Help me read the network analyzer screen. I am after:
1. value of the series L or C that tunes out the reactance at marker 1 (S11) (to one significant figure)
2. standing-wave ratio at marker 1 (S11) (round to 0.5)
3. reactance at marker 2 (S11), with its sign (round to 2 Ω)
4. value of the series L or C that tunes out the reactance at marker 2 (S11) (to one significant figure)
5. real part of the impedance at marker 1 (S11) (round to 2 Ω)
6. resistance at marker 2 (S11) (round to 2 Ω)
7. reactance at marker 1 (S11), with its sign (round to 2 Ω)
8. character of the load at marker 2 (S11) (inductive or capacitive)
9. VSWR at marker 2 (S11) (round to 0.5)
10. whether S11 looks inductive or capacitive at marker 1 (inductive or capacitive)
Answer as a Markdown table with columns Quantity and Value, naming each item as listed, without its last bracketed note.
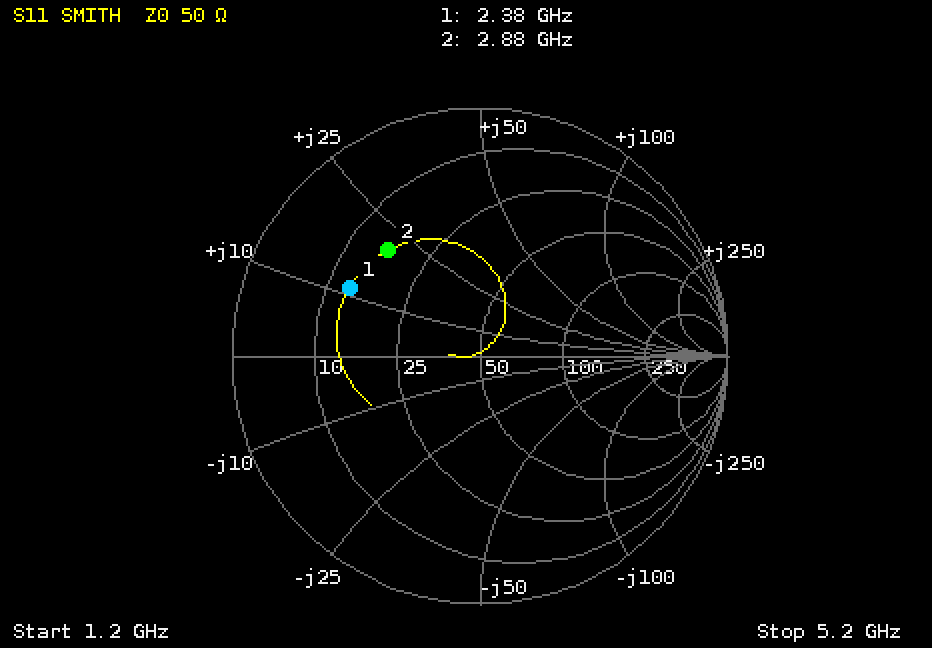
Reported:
| Quantity | Value |
|---|---|
| value of the series L or C that tunes out the reactance at marker 1 (S11) | 6 pF |
| standing-wave ratio at marker 1 (S11) | 4.0 |
| reactance at marker 2 (S11), with its sign | +20 Ω |
| value of the series L or C that tunes out the reactance at marker 2 (S11) | 3 pF |
| real part of the impedance at marker 1 (S11) | 14 Ω |
| resistance at marker 2 (S11) | 16 Ω |
| reactance at marker 1 (S11), with its sign | +12 Ω |
| character of the load at marker 2 (S11) | inductive |
| VSWR at marker 2 (S11) | 3.5 |
| whether S11 looks inductive or capacitive at marker 1 | inductive |
